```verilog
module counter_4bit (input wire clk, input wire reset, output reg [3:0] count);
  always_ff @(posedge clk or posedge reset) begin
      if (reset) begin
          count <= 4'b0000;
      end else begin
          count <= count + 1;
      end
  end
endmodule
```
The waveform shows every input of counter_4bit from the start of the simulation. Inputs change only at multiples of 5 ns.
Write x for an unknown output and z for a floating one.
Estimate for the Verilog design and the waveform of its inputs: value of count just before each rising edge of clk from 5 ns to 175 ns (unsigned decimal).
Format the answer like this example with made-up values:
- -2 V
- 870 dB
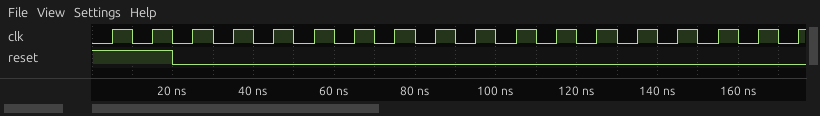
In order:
- 0, 0, 0, 1, 2, 3, 4, 5, 6, 7, 8, 9, 10, 11, 12, 13, 14, 15
